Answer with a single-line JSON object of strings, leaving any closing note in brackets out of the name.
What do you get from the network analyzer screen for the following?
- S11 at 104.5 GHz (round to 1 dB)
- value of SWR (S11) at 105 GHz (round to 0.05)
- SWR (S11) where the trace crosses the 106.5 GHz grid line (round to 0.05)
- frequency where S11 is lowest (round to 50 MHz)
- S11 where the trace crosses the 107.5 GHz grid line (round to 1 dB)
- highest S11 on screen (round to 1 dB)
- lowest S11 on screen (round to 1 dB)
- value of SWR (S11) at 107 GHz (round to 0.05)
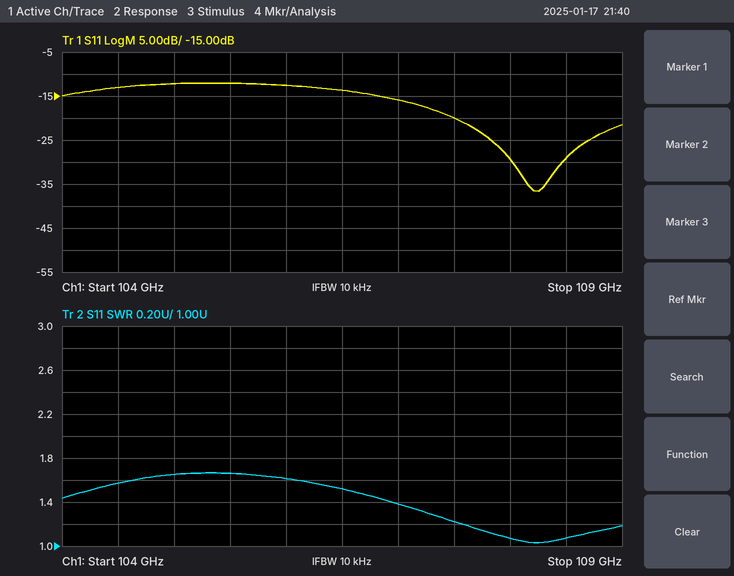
{"S11 at 104.5 GHz": "-13 dB", "value of SWR (S11) at 105 GHz": "1.65", "SWR (S11) where the trace crosses the 106.5 GHz grid line": "1.50", "frequency where S11 is lowest": "108.25 GHz", "S11 where the trace crosses the 107.5 GHz grid line": "-20 dB", "highest S11 on screen": "-12 dB", "lowest S11 on screen": "-37 dB", "value of SWR (S11) at 107 GHz": "1.40"}
